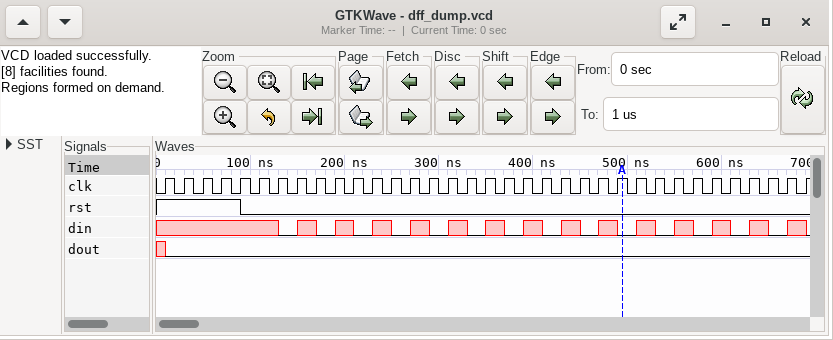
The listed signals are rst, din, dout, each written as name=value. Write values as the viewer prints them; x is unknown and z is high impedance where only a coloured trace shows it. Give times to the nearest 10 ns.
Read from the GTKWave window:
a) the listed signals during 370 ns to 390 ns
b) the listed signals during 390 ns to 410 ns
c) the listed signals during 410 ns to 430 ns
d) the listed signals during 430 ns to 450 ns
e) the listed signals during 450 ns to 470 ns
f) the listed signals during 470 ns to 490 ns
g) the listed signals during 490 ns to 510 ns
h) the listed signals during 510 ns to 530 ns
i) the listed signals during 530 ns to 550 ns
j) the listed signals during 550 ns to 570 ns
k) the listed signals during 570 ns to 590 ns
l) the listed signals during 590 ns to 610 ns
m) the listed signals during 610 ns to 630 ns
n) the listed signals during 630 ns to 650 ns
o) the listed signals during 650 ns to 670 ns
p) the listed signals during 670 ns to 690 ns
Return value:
rst=0, din=0, dout=0
rst=0, din=x, dout=0
rst=0, din=0, dout=0
rst=0, din=x, dout=0
rst=0, din=0, dout=0
rst=0, din=x, dout=0
rst=0, din=0, dout=0
rst=0, din=x, dout=0
rst=0, din=0, dout=0
rst=0, din=x, dout=0
rst=0, din=0, dout=0
rst=0, din=x, dout=0
rst=0, din=0, dout=0
rst=0, din=x, dout=0
rst=0, din=0, dout=0
rst=0, din=x, dout=0
